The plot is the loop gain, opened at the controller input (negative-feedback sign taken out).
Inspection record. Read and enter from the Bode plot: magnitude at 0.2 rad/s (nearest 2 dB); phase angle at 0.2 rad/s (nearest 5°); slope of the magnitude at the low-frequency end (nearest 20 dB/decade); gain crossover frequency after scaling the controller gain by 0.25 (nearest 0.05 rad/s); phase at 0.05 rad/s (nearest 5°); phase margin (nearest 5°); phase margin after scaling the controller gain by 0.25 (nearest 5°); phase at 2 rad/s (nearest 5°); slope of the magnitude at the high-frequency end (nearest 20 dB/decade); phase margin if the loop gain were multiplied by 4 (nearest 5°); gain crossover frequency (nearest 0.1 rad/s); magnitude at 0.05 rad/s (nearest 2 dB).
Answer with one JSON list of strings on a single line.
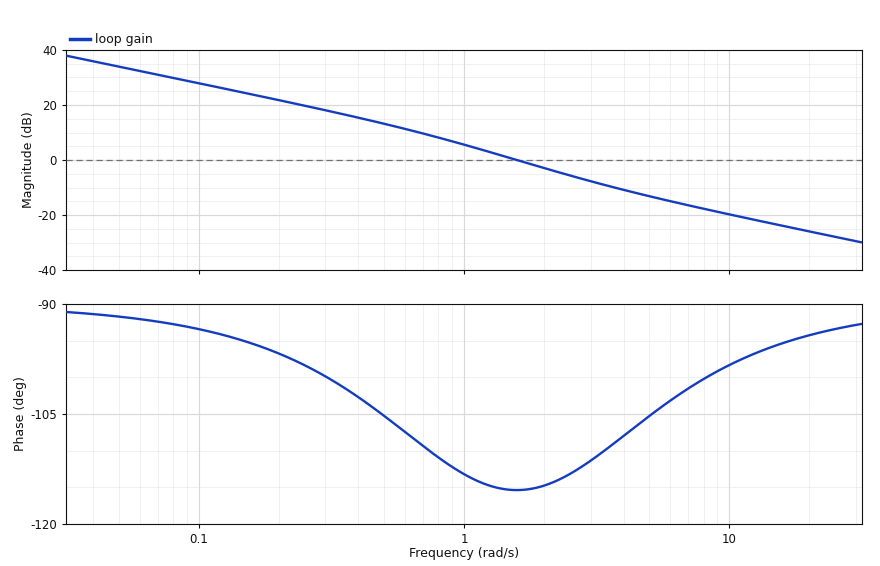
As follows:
["22 dB", "-95°", "-20 dB/decade", "0.55 rad/s", "-90°", "65°", "75°", "-115°", "-20 dB/decade", "75°", "1.6 rad/s", "34 dB"]
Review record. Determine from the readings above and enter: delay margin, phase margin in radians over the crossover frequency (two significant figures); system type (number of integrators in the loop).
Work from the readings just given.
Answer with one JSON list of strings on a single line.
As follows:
["0.71 s", "1"]
